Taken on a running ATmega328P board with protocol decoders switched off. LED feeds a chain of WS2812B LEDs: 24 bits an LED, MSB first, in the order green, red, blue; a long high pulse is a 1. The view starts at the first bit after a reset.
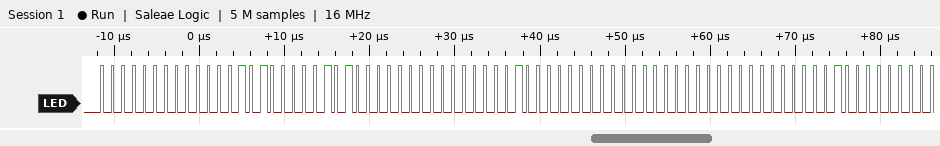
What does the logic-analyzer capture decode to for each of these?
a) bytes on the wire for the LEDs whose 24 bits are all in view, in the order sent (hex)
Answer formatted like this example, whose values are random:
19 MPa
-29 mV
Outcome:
00 05 05 00 01 00 00 00 04
